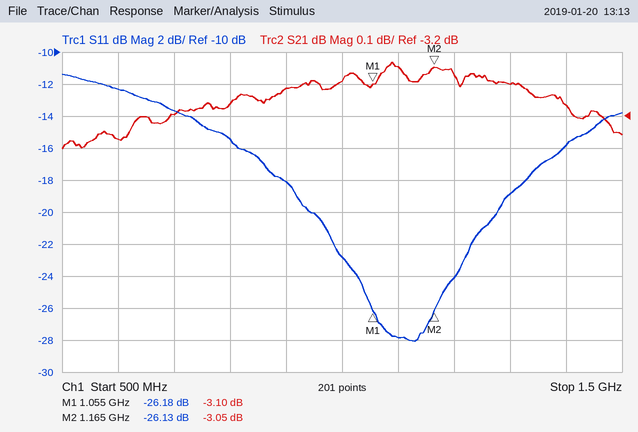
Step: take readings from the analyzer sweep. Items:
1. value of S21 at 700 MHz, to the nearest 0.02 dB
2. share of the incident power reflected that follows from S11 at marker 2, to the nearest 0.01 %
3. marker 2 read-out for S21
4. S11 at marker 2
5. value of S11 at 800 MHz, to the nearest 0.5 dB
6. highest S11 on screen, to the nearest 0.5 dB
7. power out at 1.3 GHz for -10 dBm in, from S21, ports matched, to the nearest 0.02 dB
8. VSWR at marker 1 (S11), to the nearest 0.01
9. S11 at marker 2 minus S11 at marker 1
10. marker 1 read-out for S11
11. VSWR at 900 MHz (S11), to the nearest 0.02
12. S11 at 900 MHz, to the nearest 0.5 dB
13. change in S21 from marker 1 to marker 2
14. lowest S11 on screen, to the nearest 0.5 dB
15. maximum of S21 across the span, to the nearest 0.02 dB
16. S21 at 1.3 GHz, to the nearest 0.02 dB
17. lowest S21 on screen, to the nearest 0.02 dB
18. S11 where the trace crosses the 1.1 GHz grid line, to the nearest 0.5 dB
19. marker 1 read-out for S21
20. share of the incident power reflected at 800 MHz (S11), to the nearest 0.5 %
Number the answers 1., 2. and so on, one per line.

1. -3.20 dB
2. 0.24 %
3. -3.05 dB
4. -26.13 dB
5. -15.5 dB
6. -11.5 dB
7. -13.10 dBm
8. 1.10
9. 0.05 dB
10. -26.18 dB
11. 1.28
12. -18.0 dB
13. 0.05 dB
14. -28.0 dB
15. -3.04 dB
16. -3.10 dB
17. -3.30 dB
18. -28.0 dB
19. -3.10 dB
20. 3.0 %
